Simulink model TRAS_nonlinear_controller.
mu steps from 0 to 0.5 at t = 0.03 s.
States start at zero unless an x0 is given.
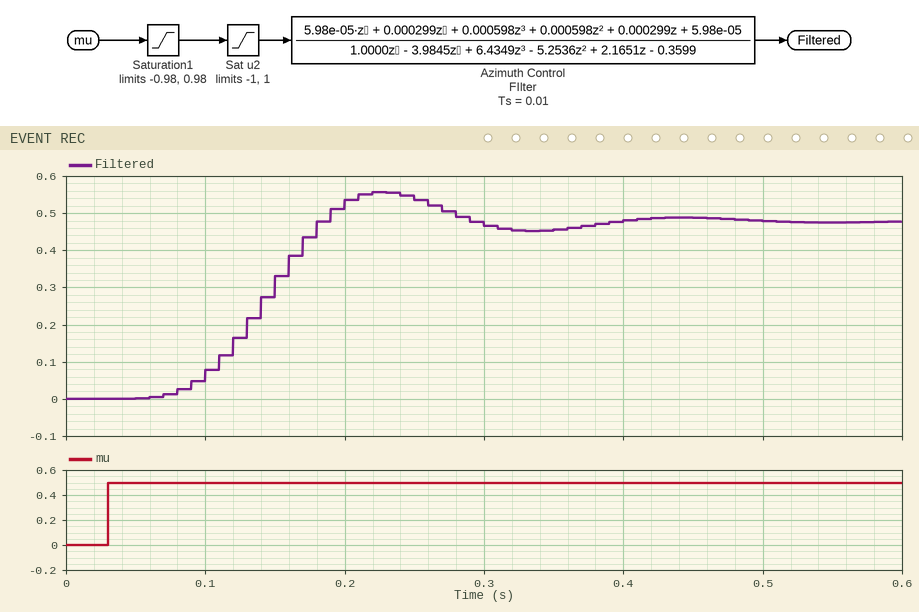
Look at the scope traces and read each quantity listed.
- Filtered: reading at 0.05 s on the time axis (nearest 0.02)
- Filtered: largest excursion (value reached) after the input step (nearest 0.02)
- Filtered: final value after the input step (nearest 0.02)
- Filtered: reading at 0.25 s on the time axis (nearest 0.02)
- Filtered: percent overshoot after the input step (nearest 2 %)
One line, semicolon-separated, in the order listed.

0.00; 0.56; 0.48; 0.54; 16 %
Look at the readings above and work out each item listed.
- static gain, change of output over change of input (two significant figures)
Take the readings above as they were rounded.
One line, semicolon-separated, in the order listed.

0.96
